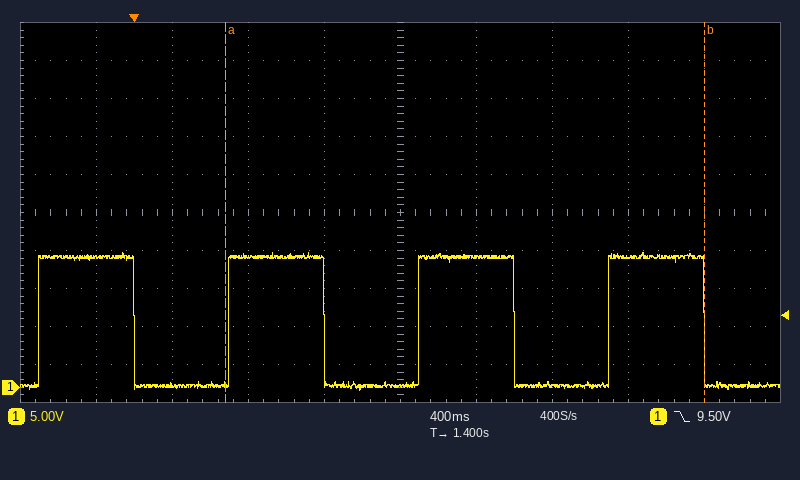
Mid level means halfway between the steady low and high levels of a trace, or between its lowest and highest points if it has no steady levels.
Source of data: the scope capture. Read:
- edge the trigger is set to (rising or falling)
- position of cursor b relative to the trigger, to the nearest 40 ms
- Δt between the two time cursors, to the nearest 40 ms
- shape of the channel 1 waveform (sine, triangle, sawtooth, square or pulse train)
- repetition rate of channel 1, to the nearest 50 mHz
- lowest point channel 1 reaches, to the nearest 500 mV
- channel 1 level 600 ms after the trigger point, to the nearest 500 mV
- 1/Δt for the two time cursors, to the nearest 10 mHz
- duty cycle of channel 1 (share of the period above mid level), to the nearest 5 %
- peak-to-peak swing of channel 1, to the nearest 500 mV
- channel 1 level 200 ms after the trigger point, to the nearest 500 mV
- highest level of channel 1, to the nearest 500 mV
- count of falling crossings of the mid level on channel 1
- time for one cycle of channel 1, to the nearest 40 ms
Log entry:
falling
+3.00 s
2.52 s
square
1.00 Hz
-500 mV
17.0 V
400 mHz
50 %
18.0 V
500 mV
17.5 V
4
1.00 s
